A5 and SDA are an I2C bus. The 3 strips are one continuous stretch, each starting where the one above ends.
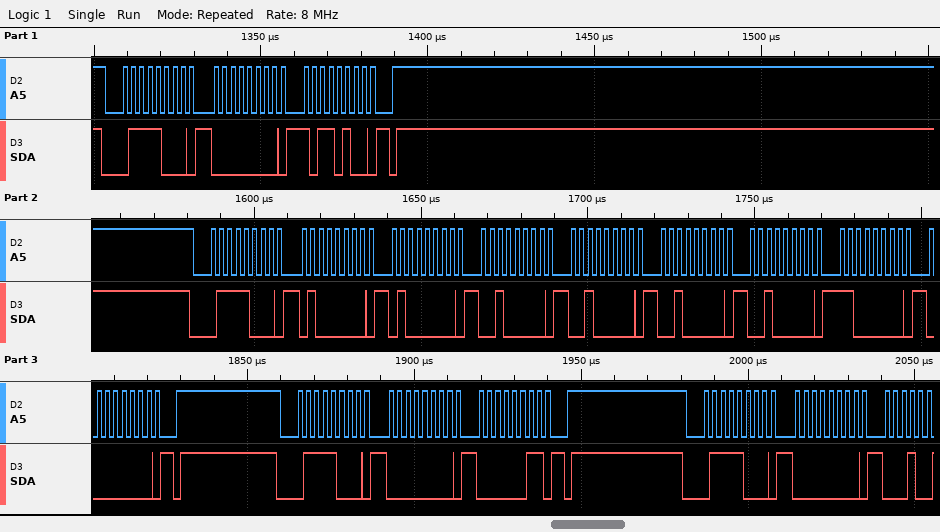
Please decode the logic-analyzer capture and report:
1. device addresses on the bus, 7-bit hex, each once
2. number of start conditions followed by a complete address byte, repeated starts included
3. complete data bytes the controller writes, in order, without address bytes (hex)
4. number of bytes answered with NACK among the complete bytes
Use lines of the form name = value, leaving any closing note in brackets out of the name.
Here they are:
device addresses on the bus, 7-bit hex, each once = 0x3C
number of start conditions followed by a complete address byte, repeated starts included = 4
complete data bytes the controller writes, in order, without address bytes = 00 B4 40 40 20 20 20 20 C0 00 00 03 00
number of bytes answered with NACK among the complete bytes = 0
